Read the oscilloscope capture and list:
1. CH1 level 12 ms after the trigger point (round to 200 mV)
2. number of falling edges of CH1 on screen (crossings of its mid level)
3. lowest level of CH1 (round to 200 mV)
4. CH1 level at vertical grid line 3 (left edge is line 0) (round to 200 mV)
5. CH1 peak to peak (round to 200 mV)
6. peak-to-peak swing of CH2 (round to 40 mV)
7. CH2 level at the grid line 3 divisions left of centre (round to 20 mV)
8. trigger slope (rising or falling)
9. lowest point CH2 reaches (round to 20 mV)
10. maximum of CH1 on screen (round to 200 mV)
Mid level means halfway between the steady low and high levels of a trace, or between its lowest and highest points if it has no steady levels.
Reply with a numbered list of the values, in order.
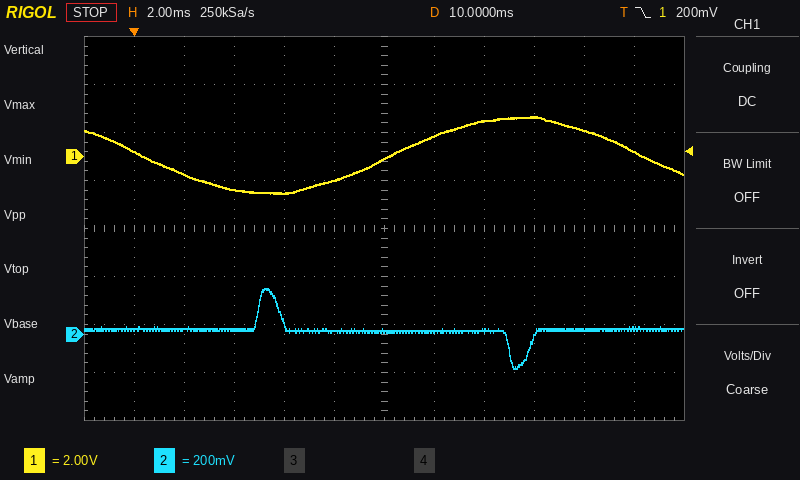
1. 800 mV
2. 2
3. -1.6 V
4. -1.4 V
5. 3.2 V
6. 320 mV
7. 20 mV
8. falling
9. -140 mV
10. 1.6 V
